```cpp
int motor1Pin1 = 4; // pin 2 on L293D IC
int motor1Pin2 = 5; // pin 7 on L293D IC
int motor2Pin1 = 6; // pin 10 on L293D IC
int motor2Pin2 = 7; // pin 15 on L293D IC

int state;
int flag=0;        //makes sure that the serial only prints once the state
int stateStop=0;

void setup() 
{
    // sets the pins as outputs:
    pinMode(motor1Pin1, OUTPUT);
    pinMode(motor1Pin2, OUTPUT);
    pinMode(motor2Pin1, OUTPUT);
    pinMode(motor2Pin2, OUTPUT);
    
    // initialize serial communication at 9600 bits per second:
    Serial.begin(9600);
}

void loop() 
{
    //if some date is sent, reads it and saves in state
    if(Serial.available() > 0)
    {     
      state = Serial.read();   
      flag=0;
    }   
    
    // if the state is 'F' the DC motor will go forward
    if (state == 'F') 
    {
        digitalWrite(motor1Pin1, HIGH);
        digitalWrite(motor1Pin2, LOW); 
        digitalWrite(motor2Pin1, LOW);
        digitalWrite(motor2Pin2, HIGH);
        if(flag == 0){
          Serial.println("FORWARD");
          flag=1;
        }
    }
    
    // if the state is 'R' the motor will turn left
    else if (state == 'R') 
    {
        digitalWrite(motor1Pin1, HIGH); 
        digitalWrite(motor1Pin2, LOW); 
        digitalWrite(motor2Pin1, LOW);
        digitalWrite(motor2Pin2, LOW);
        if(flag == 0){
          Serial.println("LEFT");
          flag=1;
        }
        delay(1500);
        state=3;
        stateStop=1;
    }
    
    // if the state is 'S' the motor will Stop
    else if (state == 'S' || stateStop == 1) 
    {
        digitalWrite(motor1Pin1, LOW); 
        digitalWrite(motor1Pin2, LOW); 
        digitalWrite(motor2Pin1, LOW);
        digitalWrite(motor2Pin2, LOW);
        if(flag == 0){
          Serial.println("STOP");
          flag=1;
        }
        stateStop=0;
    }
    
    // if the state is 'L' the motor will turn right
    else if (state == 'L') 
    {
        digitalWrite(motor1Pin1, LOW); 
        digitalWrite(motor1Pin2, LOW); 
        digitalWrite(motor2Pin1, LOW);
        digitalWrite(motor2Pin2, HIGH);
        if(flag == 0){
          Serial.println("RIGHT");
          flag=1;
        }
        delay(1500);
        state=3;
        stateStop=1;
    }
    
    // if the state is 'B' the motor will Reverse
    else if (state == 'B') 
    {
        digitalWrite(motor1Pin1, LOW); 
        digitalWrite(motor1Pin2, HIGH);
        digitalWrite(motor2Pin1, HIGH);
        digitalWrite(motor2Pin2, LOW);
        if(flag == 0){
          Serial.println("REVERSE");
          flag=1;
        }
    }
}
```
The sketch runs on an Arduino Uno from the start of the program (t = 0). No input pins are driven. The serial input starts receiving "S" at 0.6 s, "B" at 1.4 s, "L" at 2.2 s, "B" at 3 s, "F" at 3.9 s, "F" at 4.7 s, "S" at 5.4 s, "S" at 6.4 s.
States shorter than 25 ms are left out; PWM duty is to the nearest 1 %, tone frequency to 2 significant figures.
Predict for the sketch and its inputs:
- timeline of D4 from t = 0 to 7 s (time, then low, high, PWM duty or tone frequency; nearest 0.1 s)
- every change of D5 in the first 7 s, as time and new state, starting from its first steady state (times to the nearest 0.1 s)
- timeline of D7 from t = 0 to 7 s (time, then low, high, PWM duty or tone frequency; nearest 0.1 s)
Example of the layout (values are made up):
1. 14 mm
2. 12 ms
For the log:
1. 0 s low; 3.9 s high; 5.4 s low
2. 0 s low; 1.4 s high; 2.2 s low; 3.7 s high; 3.9 s low
3. 0 s low; 2.2 s high; 3.7 s low; 3.9 s high; 5.4 s low
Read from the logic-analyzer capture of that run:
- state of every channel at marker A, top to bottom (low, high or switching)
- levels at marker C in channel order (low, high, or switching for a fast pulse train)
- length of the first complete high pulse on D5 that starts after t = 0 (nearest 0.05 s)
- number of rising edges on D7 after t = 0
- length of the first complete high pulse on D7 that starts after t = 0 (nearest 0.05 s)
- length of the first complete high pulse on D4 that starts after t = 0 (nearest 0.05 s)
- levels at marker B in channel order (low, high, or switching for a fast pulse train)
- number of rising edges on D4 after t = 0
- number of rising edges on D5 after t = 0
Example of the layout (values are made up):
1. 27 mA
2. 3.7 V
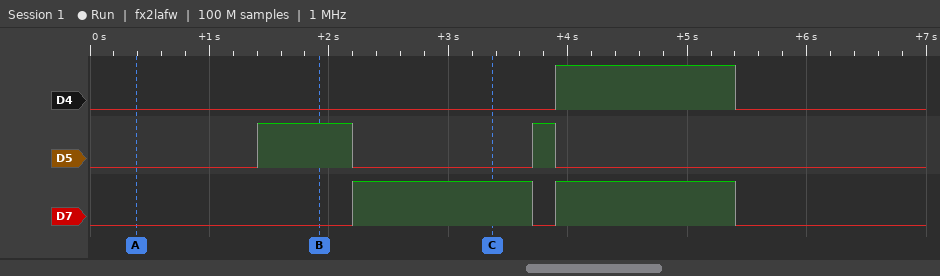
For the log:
1. D4 low, D5 low, D7 low
2. D4 low, D5 low, D7 high
3. 0.80 s
4. 2
5. 1.50 s
6. 1.50 s
7. D4 low, D5 high, D7 low
8. 1
9. 2
